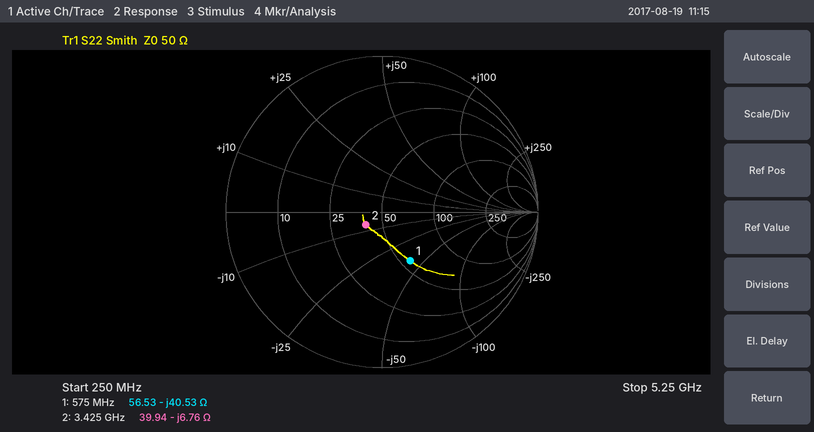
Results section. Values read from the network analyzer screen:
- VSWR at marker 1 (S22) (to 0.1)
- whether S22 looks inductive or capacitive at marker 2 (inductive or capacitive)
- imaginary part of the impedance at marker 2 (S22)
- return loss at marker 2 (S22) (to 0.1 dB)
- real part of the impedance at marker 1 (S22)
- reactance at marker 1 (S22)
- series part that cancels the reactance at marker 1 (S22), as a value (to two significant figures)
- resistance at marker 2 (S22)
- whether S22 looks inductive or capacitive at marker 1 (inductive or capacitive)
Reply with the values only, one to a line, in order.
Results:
2.1
capacitive
-6.76 Ω
17.4 dB
56.53 Ω
-40.53 Ω
11 nH
39.94 Ω
capacitive
